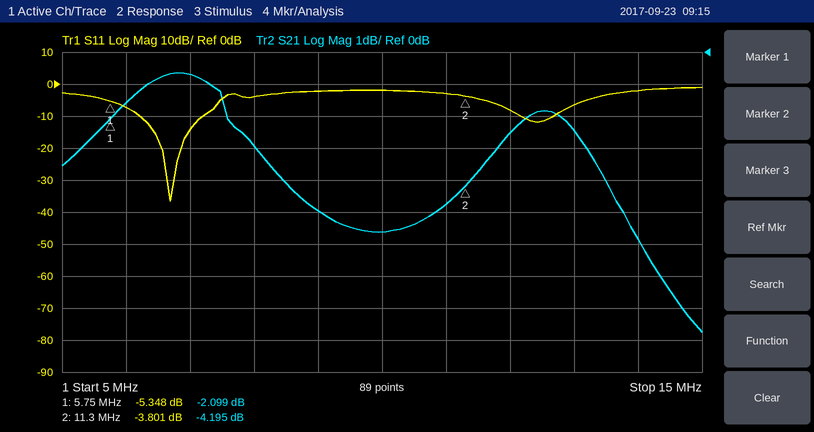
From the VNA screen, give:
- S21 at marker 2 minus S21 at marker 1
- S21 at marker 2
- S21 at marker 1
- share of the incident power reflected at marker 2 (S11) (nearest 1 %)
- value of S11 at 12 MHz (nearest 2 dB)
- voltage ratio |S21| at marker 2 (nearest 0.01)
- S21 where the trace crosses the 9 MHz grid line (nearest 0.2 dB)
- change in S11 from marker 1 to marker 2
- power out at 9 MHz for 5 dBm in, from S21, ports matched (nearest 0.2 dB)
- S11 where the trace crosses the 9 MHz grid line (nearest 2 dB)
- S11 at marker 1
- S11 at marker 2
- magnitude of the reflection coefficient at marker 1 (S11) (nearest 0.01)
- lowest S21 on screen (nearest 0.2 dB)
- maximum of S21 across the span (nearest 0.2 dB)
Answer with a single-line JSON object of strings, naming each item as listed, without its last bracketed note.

{"S21 at marker 2 minus S21 at marker 1": "-2.096 dB", "S21 at marker 2": "-4.195 dB", "S21 at marker 1": "-2.099 dB", "share of the incident power reflected at marker 2 (S11)": "42 %", "value of S11 at 12 MHz": "-8 dB", "voltage ratio |S21| at marker 2": "0.62", "S21 where the trace crosses the 9 MHz grid line": "-5.0 dB", "change in S11 from marker 1 to marker 2": "1.547 dB", "power out at 9 MHz for 5 dBm in, from S21, ports matched": "0.0 dBm", "S11 where the trace crosses the 9 MHz grid line": "-2 dB", "S11 at marker 1": "-5.348 dB", "S11 at marker 2": "-3.801 dB", "magnitude of the reflection coefficient at marker 1 (S11)": "0.54", "lowest S21 on screen": "-8.8 dB", "maximum of S21 across the span": "-0.6 dB"}
